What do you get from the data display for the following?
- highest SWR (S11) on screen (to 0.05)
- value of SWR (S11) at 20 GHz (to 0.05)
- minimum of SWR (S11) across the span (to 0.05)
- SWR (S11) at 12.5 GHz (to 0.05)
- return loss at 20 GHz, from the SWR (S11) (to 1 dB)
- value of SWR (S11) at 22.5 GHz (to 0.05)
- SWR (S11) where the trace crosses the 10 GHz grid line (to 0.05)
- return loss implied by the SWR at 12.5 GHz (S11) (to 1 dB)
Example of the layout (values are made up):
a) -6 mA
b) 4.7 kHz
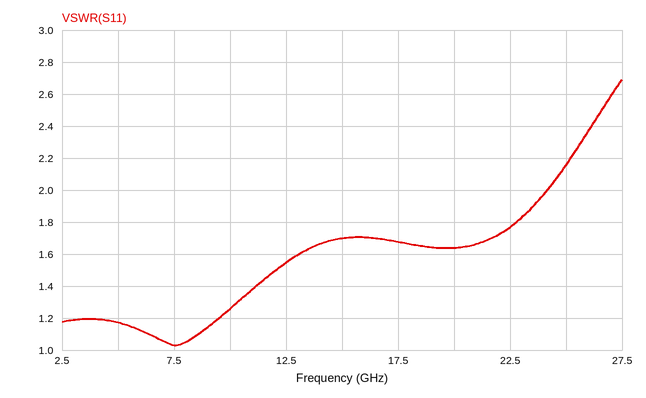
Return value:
a) 2.70
b) 1.65
c) 1.05
d) 1.55
e) 12 dB
f) 1.75
g) 1.25
h) 13 dB
